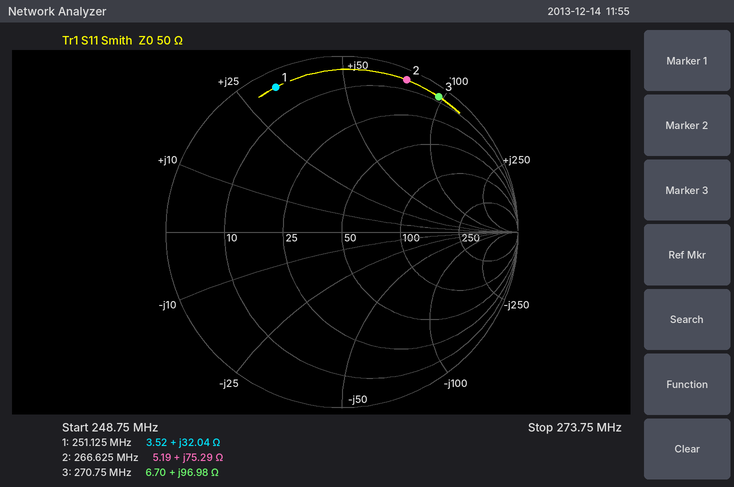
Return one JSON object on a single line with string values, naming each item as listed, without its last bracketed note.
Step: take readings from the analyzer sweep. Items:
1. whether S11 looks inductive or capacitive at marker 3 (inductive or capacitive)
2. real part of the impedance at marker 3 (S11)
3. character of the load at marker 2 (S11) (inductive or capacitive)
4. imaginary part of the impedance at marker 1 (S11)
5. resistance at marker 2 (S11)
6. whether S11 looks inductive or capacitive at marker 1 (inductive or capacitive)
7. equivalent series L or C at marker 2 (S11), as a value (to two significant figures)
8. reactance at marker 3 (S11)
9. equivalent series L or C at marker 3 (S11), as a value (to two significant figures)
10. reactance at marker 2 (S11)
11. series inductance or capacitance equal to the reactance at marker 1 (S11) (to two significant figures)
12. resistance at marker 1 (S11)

{"whether S11 looks inductive or capacitive at marker 3": "inductive", "real part of the impedance at marker 3": "6.70 Ω", "character of the load at marker 2 (S11)": "inductive", "imaginary part of the impedance at marker 1": "+32.04 Ω", "resistance at marker 2": "5.19 Ω", "whether S11 looks inductive or capacitive at marker 1": "inductive", "equivalent series L or C at marker 2 (S11), as a value": "45 nH", "reactance at marker 3": "+96.98 Ω", "equivalent series L or C at marker 3 (S11), as a value": "57 nH", "reactance at marker 2": "+75.29 Ω", "series inductance or capacitance equal to the reactance at marker 1 (S11)": "20 nH", "resistance at marker 1": "3.52 Ω"}
